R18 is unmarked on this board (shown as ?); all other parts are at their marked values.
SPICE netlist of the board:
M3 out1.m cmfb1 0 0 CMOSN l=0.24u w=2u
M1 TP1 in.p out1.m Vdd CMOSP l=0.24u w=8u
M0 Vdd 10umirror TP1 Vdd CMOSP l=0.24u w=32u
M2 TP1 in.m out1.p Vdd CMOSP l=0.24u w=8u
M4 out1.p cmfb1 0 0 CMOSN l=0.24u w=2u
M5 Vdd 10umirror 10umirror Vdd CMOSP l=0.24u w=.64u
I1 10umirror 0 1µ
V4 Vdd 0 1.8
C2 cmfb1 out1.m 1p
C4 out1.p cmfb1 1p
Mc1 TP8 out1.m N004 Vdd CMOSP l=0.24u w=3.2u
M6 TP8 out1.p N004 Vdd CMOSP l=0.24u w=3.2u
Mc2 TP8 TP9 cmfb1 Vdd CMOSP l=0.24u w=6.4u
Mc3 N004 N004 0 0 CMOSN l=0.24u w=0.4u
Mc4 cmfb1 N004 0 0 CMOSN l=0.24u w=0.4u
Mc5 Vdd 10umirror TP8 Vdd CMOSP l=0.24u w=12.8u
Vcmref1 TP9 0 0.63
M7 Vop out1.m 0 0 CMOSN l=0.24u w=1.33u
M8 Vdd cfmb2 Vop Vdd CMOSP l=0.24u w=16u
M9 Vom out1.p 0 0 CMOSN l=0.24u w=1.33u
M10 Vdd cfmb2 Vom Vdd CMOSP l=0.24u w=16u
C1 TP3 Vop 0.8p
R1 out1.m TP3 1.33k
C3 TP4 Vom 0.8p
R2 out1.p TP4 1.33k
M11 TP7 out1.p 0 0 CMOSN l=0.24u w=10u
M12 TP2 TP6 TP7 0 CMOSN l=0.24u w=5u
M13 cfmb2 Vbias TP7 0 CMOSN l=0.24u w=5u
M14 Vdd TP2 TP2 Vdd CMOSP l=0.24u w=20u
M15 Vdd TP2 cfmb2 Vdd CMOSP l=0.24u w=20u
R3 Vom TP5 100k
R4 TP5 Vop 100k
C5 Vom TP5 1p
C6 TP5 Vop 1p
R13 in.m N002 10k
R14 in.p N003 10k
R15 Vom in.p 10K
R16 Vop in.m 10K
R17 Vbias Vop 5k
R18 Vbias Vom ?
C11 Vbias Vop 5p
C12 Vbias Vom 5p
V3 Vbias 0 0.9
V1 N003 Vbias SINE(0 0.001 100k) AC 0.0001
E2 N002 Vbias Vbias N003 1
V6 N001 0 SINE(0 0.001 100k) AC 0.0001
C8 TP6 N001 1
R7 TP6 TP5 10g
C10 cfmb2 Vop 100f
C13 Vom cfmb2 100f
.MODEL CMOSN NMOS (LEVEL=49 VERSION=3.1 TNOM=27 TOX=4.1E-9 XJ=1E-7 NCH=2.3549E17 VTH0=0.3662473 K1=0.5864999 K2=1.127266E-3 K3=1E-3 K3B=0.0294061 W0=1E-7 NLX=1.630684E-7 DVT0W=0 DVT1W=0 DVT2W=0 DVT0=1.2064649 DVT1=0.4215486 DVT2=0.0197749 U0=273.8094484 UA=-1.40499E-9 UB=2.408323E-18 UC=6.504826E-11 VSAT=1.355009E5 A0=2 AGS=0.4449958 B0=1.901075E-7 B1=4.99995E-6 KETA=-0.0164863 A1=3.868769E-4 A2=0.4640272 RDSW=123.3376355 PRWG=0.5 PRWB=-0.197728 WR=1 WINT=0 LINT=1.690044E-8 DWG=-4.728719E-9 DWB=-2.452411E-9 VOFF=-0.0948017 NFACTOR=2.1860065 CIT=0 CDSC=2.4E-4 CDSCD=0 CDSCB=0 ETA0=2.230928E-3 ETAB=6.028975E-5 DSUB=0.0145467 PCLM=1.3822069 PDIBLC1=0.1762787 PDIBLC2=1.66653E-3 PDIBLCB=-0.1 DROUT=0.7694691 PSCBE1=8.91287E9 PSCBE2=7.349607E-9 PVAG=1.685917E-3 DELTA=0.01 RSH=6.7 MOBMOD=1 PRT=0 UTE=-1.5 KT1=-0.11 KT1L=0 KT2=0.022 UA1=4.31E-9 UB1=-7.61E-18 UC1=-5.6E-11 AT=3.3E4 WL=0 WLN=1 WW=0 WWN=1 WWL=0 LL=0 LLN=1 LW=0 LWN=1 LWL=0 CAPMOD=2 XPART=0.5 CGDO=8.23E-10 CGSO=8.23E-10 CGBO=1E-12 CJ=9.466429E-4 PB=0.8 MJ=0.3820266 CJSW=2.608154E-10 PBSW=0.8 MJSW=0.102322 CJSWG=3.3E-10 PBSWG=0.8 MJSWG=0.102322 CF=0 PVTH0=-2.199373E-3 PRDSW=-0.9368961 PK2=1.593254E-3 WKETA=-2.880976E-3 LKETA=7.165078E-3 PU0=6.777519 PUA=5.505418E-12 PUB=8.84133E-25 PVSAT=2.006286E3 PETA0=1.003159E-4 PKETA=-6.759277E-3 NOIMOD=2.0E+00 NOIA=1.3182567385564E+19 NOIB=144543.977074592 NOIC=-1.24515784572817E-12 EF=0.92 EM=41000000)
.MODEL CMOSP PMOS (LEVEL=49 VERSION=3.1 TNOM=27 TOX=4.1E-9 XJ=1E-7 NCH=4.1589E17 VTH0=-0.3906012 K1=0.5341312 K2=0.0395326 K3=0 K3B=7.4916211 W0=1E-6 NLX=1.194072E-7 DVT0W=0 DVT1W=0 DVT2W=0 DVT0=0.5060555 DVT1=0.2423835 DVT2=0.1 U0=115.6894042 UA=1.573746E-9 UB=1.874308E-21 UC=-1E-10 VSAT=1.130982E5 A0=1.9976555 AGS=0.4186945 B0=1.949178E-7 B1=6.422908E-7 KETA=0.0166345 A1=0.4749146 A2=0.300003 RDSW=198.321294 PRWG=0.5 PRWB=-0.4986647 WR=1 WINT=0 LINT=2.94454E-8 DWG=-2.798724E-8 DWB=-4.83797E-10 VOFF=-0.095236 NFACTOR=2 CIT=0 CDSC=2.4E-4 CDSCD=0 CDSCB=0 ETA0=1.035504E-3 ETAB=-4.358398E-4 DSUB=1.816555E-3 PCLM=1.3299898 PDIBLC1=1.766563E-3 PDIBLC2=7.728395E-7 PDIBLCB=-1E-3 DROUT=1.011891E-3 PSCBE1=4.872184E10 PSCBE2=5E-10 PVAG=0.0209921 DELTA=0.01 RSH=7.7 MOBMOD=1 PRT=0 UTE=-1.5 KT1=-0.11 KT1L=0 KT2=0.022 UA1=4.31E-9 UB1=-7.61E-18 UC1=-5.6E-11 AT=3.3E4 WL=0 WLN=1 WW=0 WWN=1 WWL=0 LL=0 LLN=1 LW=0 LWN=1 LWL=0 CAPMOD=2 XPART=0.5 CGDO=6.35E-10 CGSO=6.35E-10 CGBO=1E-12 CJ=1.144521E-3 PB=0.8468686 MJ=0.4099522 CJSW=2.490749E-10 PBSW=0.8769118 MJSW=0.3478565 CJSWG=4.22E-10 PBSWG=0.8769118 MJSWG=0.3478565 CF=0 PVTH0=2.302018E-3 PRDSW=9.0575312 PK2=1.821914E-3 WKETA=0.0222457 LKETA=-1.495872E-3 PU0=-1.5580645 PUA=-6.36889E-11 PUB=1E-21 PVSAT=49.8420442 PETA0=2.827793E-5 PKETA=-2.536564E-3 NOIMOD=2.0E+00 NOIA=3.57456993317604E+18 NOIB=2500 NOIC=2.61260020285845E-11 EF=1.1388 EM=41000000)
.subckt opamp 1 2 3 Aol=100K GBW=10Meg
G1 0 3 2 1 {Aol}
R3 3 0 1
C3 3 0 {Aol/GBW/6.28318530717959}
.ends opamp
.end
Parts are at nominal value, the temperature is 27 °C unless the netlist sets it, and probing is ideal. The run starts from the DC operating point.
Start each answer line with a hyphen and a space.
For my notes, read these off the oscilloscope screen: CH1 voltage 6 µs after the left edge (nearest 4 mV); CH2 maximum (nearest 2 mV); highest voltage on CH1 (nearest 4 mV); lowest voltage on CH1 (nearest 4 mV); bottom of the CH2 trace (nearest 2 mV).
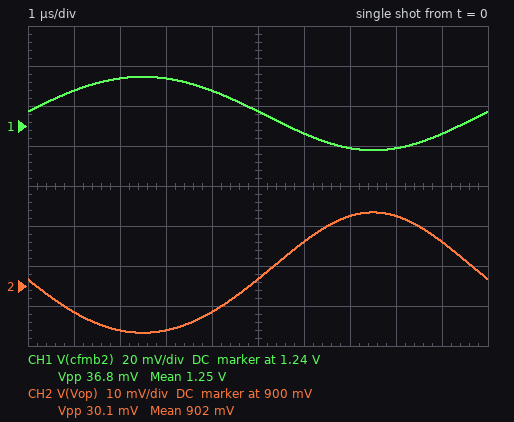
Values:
- 1.236 V
- 918 mV
- 1.264 V
- 1.228 V
- 888 mV
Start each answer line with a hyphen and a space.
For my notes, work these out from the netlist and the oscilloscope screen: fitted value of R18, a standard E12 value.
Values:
- 1.5 kΩ
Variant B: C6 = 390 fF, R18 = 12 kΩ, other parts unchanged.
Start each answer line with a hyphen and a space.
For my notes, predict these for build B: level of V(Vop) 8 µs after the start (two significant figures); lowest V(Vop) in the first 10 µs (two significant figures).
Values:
- 1.1 V
- 830 mV
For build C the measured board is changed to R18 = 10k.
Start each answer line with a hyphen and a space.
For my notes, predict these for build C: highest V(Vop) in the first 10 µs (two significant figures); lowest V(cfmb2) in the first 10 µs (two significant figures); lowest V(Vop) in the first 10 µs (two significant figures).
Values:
- 1.0 V
- 1.2 V
- 840 mV
